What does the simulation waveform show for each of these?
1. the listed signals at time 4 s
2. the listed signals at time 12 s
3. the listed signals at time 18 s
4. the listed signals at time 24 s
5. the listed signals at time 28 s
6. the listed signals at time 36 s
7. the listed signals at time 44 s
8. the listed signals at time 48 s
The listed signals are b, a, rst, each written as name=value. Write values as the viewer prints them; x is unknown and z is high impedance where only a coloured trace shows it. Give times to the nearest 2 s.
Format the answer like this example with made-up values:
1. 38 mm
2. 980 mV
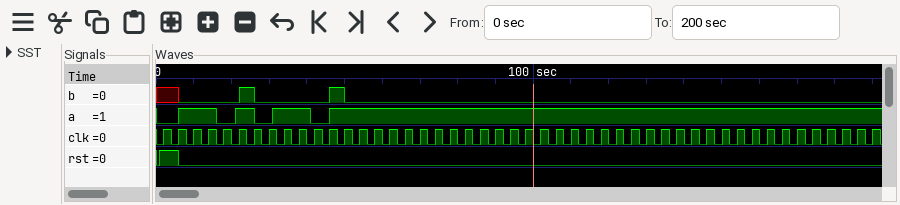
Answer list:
1. b=x, a=0, rst=1
2. b=0, a=1, rst=0
3. b=0, a=0, rst=0
4. b=1, a=1, rst=0
5. b=0, a=0, rst=0
6. b=0, a=1, rst=0
7. b=0, a=0, rst=0
8. b=1, a=1, rst=0
